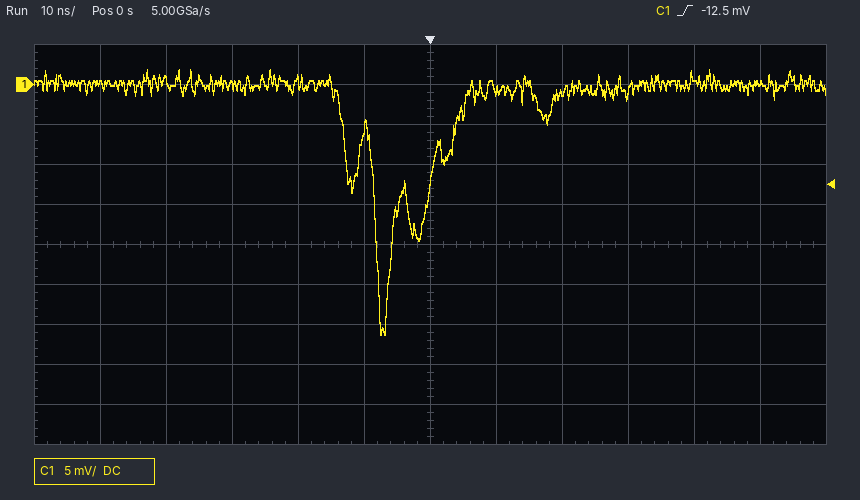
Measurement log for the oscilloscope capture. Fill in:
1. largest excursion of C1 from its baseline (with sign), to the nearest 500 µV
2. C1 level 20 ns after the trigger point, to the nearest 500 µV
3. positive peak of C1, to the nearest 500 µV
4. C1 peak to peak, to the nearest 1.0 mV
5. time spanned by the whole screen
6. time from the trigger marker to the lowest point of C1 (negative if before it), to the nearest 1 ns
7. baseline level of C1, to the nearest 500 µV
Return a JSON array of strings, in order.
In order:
["-31.0 mV", "-1.0 mV", "2.0 mV", "33.0 mV", "120 ns", "-7 ns", "0.0 mV"]
